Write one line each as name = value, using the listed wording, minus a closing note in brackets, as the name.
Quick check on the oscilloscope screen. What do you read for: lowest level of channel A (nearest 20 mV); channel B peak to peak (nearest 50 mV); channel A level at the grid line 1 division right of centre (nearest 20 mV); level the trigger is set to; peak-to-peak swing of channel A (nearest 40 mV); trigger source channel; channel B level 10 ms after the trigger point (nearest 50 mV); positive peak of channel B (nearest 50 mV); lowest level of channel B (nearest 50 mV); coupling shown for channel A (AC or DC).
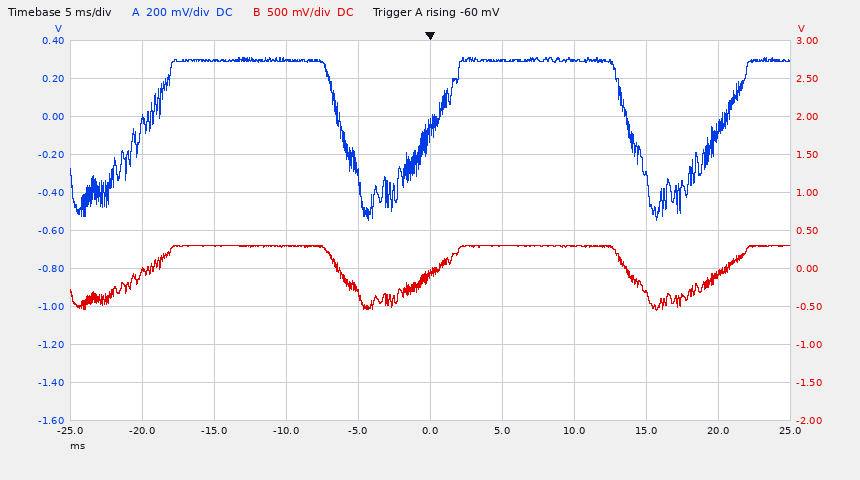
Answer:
lowest level of channel A = -540 mV
channel B peak to peak = 850 mV
channel A level at the grid line 1 division right of centre = 300 mV
level the trigger is set to = -60 mV
peak-to-peak swing of channel A = 840 mV
trigger source channel = channel A
channel B level 10 ms after the trigger point = 300 mV
positive peak of channel B = 300 mV
lowest level of channel B = -550 mV
coupling shown for channel A = DC
